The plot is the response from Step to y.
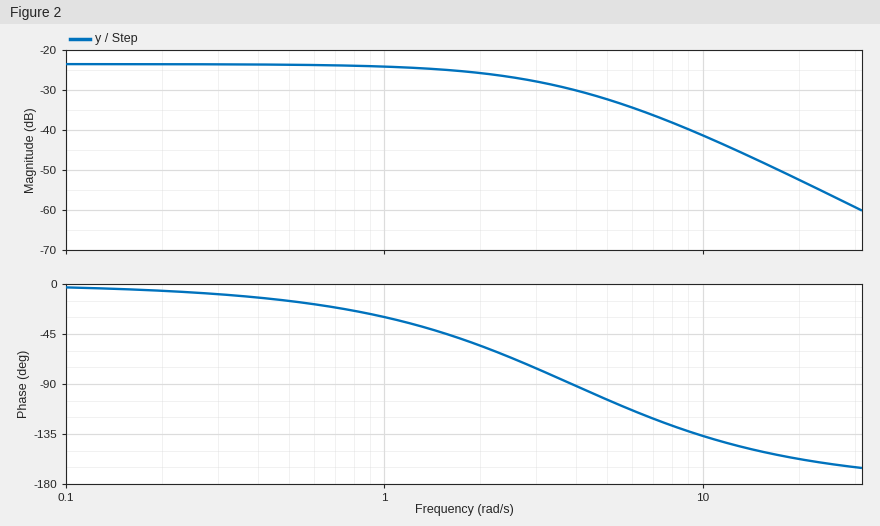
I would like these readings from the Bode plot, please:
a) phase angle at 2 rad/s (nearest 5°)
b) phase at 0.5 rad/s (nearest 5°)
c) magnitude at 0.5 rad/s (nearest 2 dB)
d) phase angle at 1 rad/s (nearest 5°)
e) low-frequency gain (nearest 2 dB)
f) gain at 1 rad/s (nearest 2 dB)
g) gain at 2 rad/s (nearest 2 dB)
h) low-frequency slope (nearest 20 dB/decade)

-55°
-15°
-24 dB
-30°
-24 dB
-24 dB
-26 dB
0 dB/decade
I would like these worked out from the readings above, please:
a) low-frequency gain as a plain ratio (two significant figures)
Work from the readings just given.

0.063
